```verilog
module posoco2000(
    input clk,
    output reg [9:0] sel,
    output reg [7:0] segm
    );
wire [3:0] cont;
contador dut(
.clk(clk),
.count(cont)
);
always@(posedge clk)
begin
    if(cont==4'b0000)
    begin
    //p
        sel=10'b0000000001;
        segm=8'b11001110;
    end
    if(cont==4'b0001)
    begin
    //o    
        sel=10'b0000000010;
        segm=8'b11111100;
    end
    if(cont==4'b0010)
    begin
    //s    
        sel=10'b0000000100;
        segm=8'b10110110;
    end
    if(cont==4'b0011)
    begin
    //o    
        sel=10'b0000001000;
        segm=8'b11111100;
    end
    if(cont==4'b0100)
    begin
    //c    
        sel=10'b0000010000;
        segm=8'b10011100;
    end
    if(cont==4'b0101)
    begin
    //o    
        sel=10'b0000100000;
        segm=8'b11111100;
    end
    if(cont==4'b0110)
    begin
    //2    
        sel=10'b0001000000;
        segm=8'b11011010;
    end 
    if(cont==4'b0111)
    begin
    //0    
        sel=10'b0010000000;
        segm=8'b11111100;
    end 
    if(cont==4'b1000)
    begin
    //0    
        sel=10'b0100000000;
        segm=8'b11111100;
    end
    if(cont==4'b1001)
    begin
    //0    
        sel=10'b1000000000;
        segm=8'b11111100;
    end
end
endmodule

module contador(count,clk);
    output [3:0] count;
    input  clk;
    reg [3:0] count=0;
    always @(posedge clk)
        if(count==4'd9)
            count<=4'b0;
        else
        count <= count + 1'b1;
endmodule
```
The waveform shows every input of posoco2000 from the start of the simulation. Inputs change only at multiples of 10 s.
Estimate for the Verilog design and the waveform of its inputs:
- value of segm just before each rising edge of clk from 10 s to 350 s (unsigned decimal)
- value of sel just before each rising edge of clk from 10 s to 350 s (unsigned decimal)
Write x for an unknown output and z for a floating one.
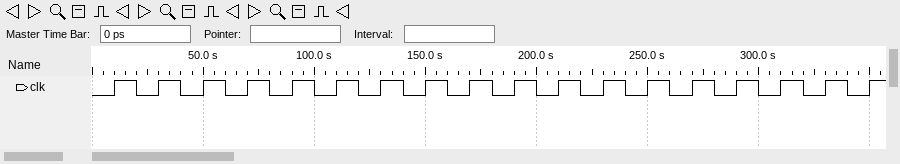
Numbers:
x, 206, 252, 182, 252, 156, 252, 218, 252, 252, 252, 206, 252, 182, 252, 156, 252, 218
x, 1, 2, 4, 8, 16, 32, 64, 128, 256, 512, 1, 2, 4, 8, 16, 32, 64
